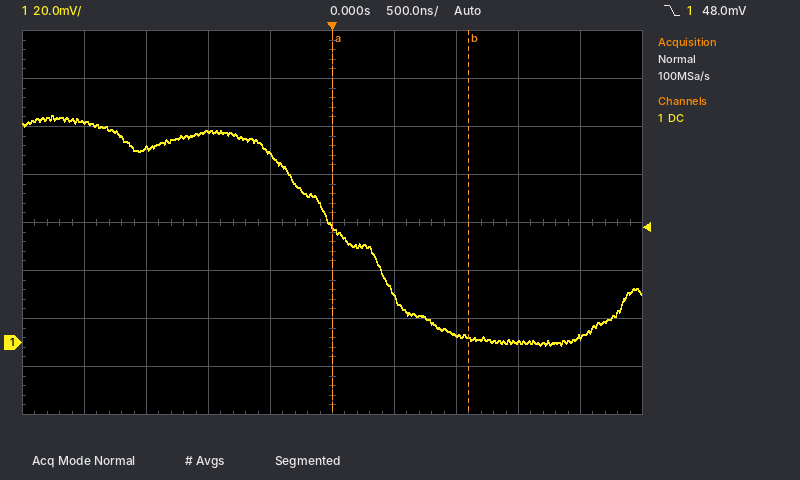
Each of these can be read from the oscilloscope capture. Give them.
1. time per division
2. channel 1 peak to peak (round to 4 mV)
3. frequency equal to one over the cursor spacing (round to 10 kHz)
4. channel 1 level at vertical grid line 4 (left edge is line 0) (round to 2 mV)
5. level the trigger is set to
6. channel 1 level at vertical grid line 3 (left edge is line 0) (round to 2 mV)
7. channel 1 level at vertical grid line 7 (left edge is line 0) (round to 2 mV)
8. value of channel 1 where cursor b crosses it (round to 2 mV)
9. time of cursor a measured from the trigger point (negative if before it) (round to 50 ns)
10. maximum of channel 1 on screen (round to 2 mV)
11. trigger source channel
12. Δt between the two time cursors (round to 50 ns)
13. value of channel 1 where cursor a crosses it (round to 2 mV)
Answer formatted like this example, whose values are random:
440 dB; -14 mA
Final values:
500 ns; 96 mV; 910 kHz; 78 mV; 48.0 mV; 88 mV; 4 mV; 2 mV; 0 ns; 94 mV; channel 1; 1.10 µs; 48 mV
